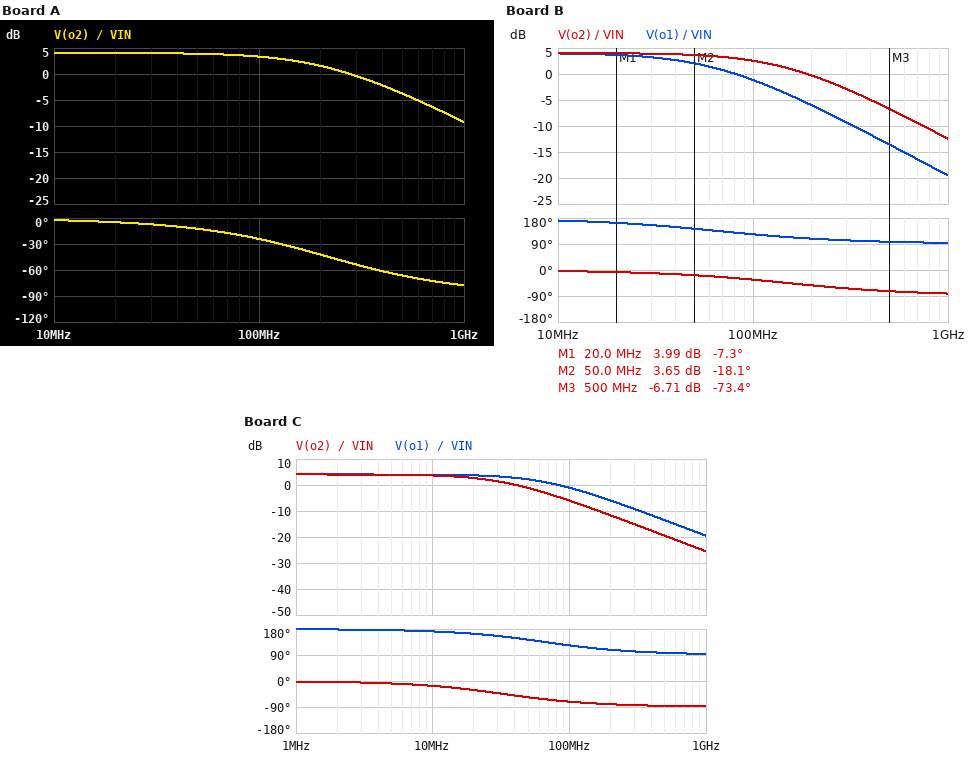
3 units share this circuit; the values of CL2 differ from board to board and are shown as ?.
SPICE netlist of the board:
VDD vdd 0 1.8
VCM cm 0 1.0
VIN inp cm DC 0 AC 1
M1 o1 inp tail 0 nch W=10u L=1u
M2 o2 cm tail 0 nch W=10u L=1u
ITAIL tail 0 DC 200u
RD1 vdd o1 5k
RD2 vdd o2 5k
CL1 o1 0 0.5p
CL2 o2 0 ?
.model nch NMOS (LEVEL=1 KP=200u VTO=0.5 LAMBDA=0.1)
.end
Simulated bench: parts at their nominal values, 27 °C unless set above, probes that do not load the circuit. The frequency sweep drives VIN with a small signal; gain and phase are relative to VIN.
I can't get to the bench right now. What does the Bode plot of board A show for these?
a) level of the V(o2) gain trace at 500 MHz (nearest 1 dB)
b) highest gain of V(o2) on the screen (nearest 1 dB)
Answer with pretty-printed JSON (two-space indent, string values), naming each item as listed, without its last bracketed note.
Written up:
{
  "level of the V(o2) gain trace at 500 MHz": "-4 dB",
  "highest gain of V(o2) on the screen": "4 dB"
}
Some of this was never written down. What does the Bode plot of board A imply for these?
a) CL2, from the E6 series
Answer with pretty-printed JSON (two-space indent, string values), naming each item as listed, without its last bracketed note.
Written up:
{
  "CL2, from the E6 series": "150 fF"
}
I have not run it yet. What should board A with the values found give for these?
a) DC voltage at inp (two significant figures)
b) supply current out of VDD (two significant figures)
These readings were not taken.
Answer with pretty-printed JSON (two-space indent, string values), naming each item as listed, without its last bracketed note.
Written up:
{
  "DC voltage at inp": "1.0 V",
  "supply current out of VDD": "200 µA"
}
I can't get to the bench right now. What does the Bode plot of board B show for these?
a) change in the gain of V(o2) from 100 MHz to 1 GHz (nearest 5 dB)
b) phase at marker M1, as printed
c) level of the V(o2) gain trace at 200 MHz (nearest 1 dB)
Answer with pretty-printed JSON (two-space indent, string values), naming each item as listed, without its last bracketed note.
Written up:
{
  "change in the gain of V(o2) from 100 MHz to 1 GHz": "-15 dB",
  "phase at marker M1, as printed": "-7.3 deg",
  "level of the V(o2) gain trace at 200 MHz": "0 dB"
}
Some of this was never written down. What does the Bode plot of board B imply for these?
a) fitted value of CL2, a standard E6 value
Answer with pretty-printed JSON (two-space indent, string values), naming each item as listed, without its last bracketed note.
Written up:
{
  "fitted value of CL2, a standard E6 value": "220 fF"
}
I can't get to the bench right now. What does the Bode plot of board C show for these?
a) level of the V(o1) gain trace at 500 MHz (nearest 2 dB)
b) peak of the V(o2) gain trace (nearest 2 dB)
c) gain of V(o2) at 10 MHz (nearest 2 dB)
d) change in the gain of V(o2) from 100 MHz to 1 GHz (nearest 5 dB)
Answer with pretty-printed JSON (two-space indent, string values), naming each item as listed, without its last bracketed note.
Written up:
{
  "level of the V(o1) gain trace at 500 MHz": "-14 dB",
  "peak of the V(o2) gain trace": "4 dB",
  "gain of V(o2) at 10 MHz": "4 dB",
  "change in the gain of V(o2) from 100 MHz to 1 GHz": "-20 dB"
}
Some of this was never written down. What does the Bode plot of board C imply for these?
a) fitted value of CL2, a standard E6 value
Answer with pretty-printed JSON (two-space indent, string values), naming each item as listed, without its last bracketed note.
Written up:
{
  "fitted value of CL2, a standard E6 value": "1 pF"
}
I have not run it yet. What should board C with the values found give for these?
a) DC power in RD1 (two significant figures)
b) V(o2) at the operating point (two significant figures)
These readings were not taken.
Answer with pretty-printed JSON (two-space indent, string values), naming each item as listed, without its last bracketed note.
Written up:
{
  "DC power in RD1": "50 µW",
  "V(o2) at the operating point": "1.3 V"
}
